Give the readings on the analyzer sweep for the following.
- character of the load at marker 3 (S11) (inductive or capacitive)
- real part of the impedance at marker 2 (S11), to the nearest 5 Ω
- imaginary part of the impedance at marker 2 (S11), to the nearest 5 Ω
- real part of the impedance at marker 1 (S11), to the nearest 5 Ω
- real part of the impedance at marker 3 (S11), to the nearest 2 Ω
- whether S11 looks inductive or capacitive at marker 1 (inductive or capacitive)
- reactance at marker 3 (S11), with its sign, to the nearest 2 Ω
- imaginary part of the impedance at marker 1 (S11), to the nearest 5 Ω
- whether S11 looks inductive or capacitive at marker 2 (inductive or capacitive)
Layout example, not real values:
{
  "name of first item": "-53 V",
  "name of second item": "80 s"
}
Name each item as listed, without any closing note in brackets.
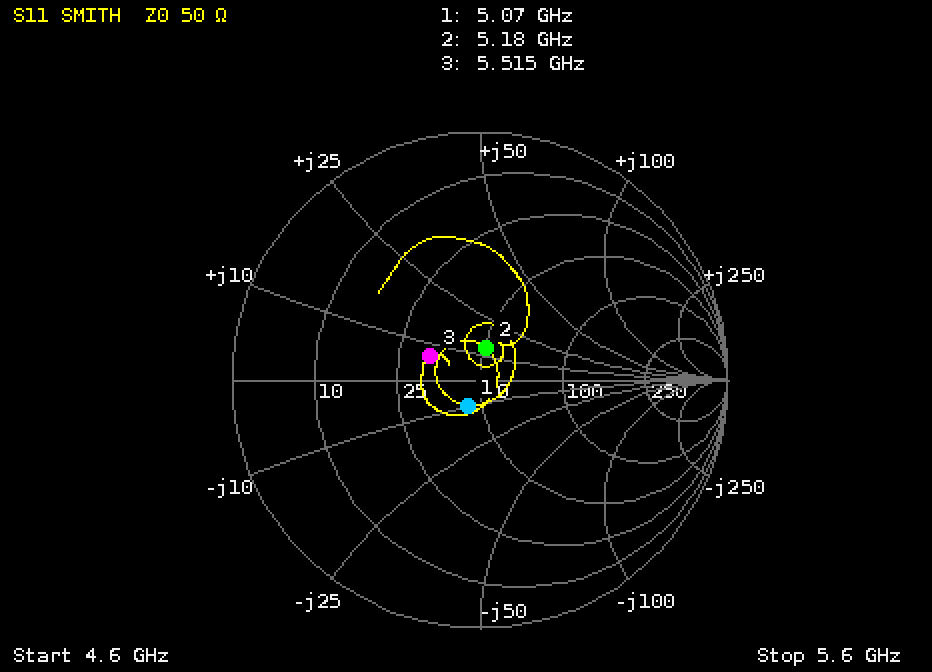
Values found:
{
  "character of the load at marker 3 (S11)": "inductive",
  "real part of the impedance at marker 2 (S11), to the nearest 5 Ω": "50 Ω",
  "imaginary part of the impedance at marker 2 (S11), to the nearest 5 Ω": "+15 Ω",
  "real part of the impedance at marker 1 (S11), to the nearest 5 Ω": "45 Ω",
  "real part of the impedance at marker 3 (S11), to the nearest 2 Ω": "32 Ω",
  "whether S11 looks inductive or capacitive at marker 1": "capacitive",
  "reactance at marker 3 (S11), with its sign, to the nearest 2 Ω": "+6 Ω",
  "imaginary part of the impedance at marker 1 (S11), to the nearest 5 Ω": "-10 Ω",
  "whether S11 looks inductive or capacitive at marker 2": "inductive"
}
